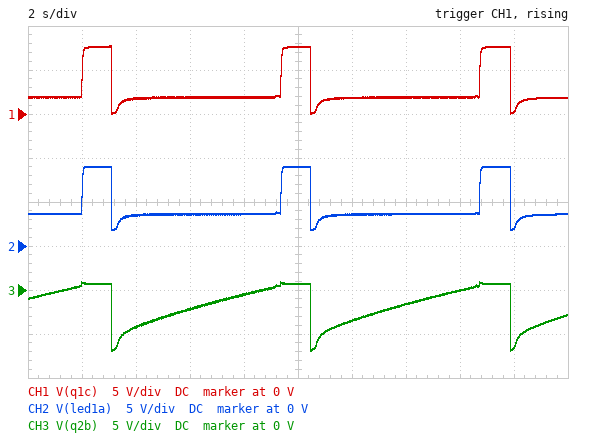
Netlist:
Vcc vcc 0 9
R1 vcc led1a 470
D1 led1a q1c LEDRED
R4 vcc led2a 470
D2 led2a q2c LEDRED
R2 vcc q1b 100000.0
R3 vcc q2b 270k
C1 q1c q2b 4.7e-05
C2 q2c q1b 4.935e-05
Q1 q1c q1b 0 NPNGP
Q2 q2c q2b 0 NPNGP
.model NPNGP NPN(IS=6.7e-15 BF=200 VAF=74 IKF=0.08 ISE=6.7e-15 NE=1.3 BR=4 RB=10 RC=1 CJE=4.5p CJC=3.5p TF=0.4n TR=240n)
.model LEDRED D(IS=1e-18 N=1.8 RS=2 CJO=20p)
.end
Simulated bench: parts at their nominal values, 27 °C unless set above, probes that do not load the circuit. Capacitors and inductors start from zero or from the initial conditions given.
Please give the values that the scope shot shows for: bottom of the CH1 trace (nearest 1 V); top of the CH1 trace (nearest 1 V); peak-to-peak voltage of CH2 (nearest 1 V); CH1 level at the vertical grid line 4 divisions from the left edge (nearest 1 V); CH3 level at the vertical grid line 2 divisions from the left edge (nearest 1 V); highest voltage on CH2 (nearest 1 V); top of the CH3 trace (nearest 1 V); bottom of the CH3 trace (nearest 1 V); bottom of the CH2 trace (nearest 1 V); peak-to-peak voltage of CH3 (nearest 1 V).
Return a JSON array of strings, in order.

["0 V", "8 V", "7 V", "2 V", "-4 V", "9 V", "1 V", "-7 V", "2 V", "8 V"]
